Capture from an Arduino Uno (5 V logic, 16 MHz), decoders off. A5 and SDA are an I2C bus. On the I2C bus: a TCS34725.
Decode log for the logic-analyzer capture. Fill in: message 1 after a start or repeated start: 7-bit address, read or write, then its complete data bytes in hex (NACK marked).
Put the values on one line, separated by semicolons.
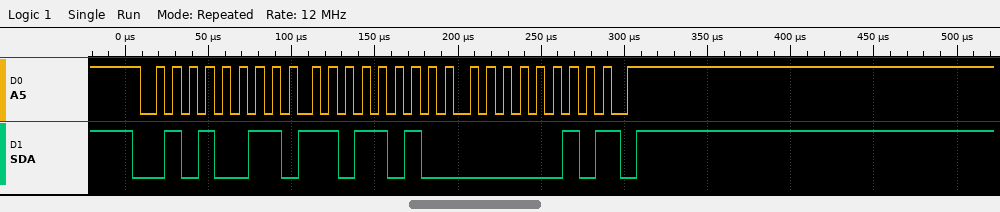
0x29 read: DA 02 NACK
